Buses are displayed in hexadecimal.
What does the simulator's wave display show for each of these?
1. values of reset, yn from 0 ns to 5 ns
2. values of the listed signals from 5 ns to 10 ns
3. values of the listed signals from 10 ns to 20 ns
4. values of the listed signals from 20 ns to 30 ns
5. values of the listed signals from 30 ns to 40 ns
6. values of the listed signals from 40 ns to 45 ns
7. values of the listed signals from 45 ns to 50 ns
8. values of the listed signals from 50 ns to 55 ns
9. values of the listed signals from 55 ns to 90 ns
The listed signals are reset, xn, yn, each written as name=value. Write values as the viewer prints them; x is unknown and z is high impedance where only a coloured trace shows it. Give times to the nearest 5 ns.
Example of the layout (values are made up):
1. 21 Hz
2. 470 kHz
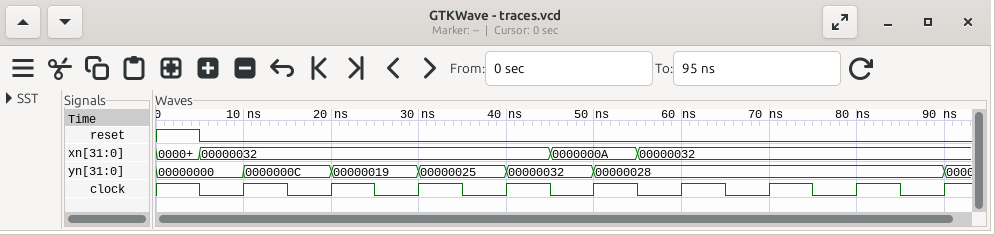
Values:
1. reset=1, yn=00000000
2. reset=0, xn=00000032, yn=00000000
3. reset=0, xn=00000032, yn=0000000C
4. reset=0, xn=00000032, yn=00000019
5. reset=0, xn=00000032, yn=00000025
6. reset=0, xn=00000032, yn=00000032
7. reset=0, xn=0000000A, yn=00000032
8. reset=0, xn=0000000A, yn=00000028
9. reset=0, xn=00000032, yn=00000028
